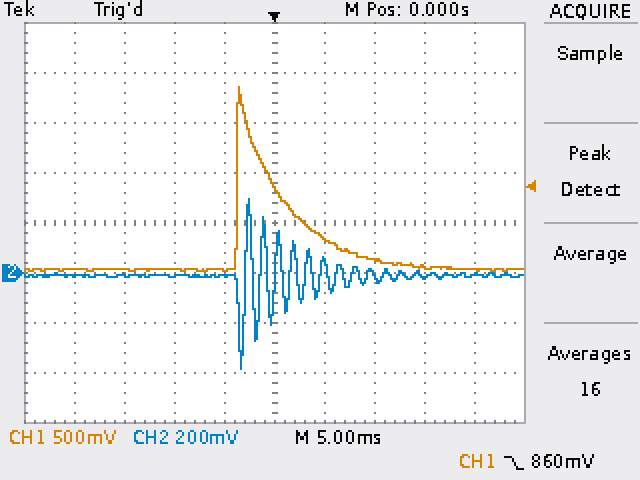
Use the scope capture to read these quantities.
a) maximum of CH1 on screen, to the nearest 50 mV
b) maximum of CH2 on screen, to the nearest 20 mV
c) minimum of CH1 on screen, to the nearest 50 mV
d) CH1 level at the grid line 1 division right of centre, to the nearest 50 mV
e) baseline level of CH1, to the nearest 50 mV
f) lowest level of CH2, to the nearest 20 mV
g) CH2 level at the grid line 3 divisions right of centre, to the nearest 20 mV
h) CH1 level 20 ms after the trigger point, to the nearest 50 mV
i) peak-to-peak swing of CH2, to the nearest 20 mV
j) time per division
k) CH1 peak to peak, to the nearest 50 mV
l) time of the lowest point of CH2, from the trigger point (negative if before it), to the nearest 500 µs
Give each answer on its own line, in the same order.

1.85 V
300 mV
0 mV
350 mV
50 mV
-380 mV
-20 mV
50 mV
680 mV
5 ms
1.85 V
-3.5 ms
